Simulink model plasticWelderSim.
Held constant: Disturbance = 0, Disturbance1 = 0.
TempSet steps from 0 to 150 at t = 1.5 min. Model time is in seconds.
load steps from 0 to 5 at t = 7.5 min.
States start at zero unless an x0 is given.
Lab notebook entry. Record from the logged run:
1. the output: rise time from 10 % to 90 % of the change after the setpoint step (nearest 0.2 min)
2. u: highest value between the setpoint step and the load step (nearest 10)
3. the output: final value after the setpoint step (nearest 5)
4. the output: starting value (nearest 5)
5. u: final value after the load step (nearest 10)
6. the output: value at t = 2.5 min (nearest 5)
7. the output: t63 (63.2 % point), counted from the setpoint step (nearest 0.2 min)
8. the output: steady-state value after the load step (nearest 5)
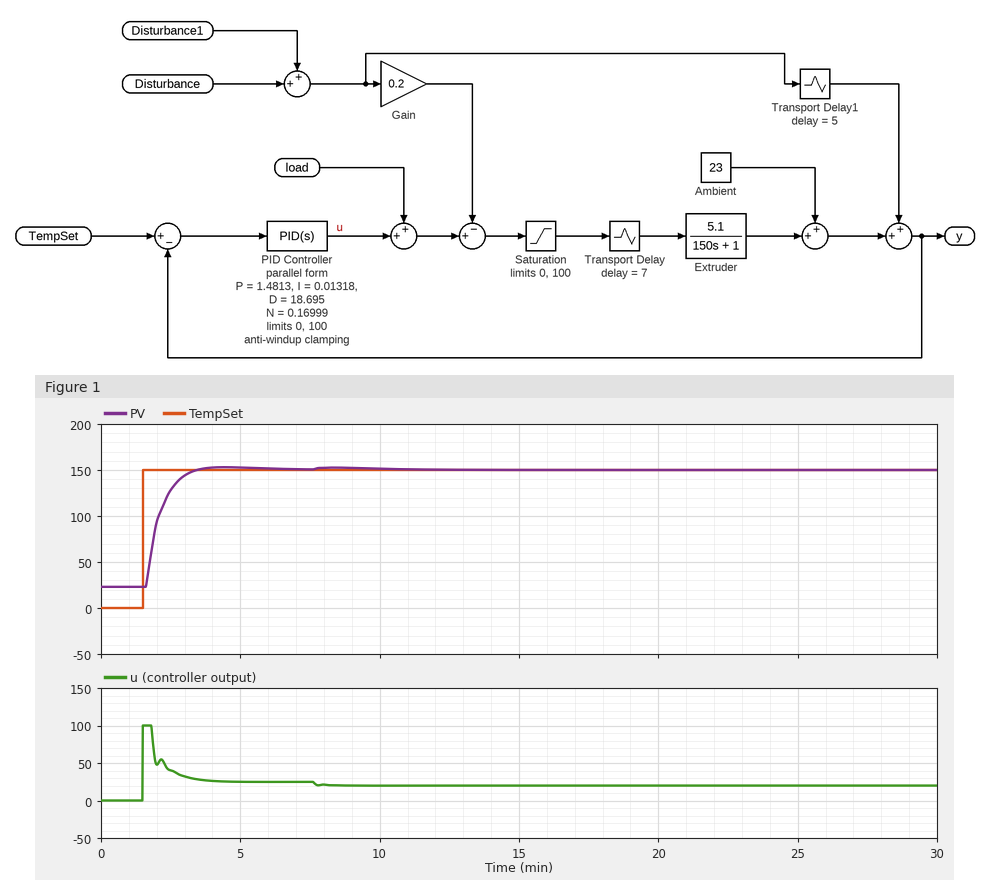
1.0 min
100
150
25
20
130
0.6 min
150
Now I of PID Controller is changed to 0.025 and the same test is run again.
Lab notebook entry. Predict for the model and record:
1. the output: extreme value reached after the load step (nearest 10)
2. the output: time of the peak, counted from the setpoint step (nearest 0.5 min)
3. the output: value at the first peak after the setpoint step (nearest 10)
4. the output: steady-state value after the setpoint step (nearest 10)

150
2.0 min
160
150
